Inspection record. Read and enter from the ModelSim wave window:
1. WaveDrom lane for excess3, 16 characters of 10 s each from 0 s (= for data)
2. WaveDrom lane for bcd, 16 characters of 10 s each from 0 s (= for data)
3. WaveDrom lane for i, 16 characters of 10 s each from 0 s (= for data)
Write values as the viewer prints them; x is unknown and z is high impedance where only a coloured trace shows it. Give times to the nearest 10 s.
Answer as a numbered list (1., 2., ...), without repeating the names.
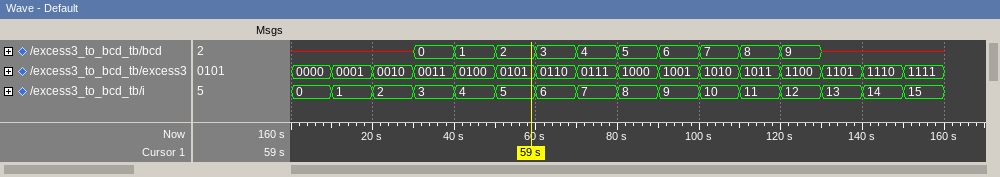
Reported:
1. {name: 'excess3', wave: '================', data: '0000 0001 0010 0011 0100 0101 0110 0111 1000 1001 1010 1011 1100 1101 1110 1111'}
2. {name: 'bcd', wave: 'x..==========x..', data: '0 1 2 3 4 5 6 7 8 9'}
3. {name: 'i', wave: '================', data: '0 1 2 3 4 5 6 7 8 9 10 11 12 13 14 15'}
